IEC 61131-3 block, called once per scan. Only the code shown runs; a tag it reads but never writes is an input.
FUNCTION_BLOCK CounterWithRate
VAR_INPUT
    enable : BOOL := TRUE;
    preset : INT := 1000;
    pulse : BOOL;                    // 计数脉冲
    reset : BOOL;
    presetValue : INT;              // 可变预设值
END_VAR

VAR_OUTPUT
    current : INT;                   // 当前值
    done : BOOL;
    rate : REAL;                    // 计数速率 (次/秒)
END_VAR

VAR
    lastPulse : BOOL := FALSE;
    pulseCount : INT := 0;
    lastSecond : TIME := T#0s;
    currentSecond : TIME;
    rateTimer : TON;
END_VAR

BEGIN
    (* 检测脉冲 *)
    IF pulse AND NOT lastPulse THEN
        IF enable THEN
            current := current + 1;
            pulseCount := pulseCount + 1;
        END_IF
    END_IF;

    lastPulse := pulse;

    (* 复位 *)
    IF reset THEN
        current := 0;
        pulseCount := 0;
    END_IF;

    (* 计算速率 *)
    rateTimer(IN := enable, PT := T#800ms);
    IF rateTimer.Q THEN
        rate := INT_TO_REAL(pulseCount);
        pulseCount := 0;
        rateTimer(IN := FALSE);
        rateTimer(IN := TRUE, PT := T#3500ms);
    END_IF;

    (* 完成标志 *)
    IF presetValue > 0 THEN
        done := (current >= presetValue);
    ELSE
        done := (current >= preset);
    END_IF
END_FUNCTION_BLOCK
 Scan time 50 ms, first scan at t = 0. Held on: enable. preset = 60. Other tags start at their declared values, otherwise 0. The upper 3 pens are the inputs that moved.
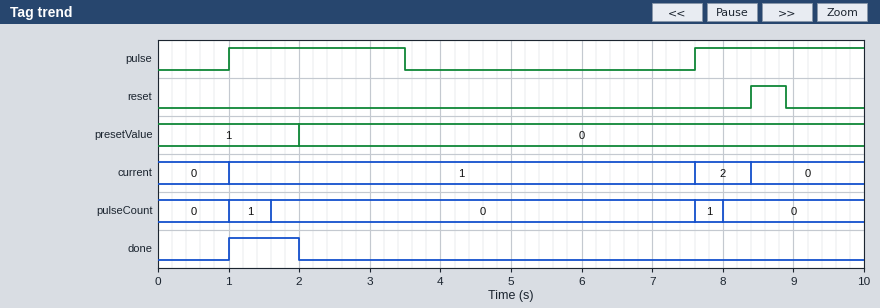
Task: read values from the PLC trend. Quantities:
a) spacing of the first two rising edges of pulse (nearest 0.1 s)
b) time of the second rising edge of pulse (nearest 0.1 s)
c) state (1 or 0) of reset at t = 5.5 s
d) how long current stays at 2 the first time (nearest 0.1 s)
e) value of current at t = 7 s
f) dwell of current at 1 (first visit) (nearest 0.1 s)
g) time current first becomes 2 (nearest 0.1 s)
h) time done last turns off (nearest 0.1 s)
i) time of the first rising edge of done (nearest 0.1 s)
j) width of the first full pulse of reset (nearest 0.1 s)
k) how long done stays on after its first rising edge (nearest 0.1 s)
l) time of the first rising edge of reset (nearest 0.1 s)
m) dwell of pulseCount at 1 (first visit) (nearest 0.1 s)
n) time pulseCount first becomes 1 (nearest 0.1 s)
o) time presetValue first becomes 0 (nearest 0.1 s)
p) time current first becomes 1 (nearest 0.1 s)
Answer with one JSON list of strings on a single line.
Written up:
["6.6 s", "7.6 s", "0", "0.8 s", "1", "6.6 s", "7.6 s", "2.0 s", "1.0 s", "0.5 s", "1.0 s", "8.4 s", "0.6 s", "1.0 s", "2.0 s", "1.0 s"]
